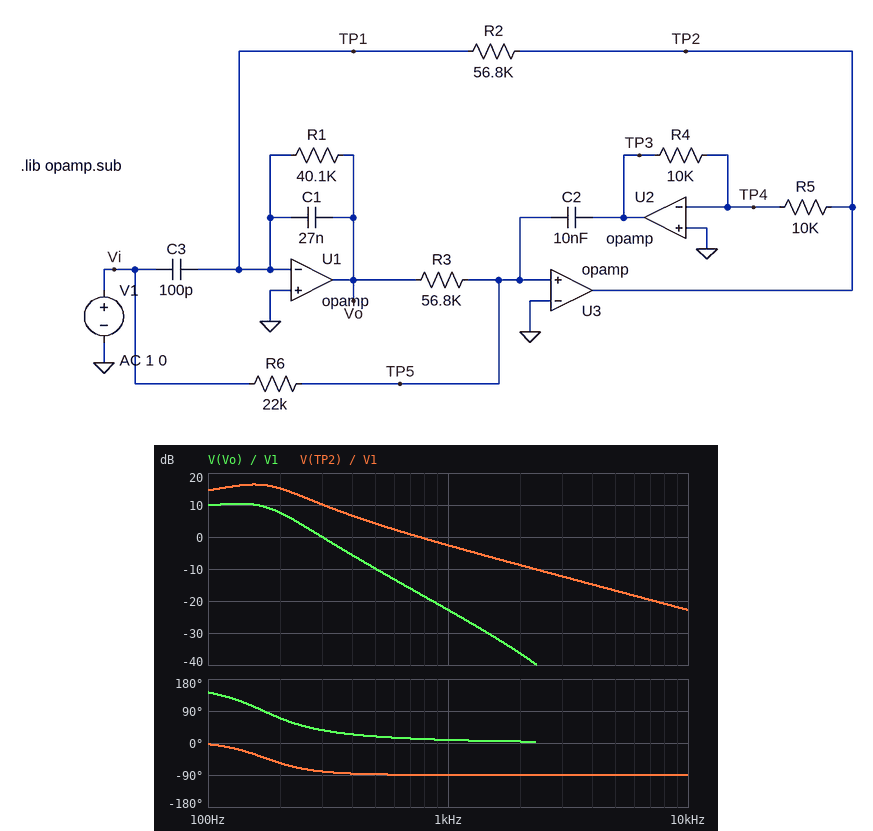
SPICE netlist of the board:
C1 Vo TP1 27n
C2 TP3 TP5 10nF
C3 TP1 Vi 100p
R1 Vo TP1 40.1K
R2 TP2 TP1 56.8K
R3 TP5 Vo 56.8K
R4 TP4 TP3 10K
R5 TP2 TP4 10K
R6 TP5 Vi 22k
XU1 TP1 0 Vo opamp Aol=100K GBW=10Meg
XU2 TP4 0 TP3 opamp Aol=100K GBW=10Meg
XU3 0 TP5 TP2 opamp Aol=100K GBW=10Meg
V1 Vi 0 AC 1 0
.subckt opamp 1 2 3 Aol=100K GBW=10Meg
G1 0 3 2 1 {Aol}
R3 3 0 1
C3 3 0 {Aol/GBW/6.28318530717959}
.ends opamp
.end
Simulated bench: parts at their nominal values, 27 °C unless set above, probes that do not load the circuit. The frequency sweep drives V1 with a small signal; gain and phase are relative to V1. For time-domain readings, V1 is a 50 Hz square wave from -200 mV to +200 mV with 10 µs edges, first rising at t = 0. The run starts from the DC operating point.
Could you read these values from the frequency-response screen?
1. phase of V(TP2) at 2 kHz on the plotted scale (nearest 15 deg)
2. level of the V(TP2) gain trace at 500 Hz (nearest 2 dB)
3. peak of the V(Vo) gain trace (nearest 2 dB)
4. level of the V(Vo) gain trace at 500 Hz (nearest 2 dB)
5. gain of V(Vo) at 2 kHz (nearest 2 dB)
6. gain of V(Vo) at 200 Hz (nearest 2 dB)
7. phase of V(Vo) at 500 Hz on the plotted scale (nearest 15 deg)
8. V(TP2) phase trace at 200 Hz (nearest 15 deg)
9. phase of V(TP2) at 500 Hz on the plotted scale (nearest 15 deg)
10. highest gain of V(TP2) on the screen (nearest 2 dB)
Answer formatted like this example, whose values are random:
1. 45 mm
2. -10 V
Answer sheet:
1. -90 deg
2. 4 dB
3. 10 dB
4. -10 dB
5. -36 dB
6. 8 dB
7. 15 deg
8. -60 deg
9. -90 deg
10. 16 dB
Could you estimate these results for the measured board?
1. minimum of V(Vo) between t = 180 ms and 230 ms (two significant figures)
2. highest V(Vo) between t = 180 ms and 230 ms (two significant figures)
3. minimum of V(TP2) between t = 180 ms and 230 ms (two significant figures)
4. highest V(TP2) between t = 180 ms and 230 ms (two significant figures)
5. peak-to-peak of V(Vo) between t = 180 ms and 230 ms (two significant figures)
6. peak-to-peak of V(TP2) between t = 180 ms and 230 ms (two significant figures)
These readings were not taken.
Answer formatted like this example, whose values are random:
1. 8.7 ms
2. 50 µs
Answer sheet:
1. -750 mV
2. 750 mV
3. -1.4 V
4. 1.4 V
5. 1.5 V
6. 2.8 V
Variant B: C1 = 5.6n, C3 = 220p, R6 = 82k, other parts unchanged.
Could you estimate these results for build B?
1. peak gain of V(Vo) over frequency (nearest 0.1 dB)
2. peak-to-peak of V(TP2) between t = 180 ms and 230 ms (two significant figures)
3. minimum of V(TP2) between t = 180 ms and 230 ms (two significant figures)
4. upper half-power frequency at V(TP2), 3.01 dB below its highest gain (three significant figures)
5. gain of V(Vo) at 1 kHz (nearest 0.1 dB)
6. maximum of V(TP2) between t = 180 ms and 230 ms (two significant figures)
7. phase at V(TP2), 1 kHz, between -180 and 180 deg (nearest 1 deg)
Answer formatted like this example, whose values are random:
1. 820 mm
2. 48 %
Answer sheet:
1. -3.2 dB
2. 390 mV
3. -200 mV
4. 289 Hz
5. -25.7 dB
6. 200 mV
7. -87 deg
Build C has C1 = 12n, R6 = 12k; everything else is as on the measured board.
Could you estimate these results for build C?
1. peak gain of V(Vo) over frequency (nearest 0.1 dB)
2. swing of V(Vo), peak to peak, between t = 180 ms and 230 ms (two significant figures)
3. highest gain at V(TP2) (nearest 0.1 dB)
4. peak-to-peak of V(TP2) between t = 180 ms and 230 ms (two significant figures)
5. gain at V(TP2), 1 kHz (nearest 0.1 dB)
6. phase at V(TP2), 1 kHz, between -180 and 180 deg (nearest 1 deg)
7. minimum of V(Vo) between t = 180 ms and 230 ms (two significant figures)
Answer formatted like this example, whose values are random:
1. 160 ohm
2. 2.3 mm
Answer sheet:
1. 13.6 dB
2. 2.2 V
3. 17.3 dB
4. 3.3 V
5. 3.0 dB
6. -89 deg
7. -1.1 V
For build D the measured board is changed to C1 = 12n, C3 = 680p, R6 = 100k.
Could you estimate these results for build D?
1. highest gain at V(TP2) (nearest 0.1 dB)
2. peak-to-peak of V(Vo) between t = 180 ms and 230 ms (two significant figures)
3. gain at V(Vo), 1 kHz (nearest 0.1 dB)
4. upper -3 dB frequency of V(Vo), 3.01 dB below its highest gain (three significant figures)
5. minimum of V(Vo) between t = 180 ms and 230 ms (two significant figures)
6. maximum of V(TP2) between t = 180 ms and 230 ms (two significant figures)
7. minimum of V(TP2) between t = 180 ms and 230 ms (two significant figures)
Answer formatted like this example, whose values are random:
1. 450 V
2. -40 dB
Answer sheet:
1. -1.2 dB
2. 260 mV
3. -34.1 dB
4. 252 Hz
5. -130 mV
6. 190 mV
7. -190 mV
